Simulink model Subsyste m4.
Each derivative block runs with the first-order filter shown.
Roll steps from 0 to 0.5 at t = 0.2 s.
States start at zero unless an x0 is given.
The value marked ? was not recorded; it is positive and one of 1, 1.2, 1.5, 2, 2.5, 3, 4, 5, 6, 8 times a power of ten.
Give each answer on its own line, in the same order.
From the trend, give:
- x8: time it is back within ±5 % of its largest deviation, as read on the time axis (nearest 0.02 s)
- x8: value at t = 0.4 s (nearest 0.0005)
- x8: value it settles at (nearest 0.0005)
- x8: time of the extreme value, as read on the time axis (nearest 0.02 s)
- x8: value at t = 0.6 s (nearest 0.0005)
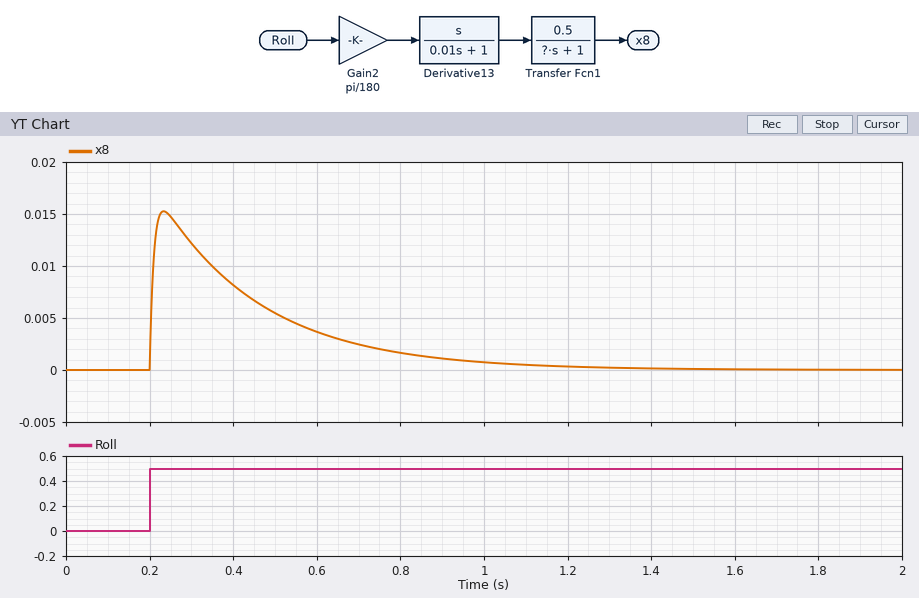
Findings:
1.00 s
0.0080
0.0000
0.24 s
0.0035
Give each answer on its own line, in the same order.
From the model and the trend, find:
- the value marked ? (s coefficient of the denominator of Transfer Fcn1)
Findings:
0.25
